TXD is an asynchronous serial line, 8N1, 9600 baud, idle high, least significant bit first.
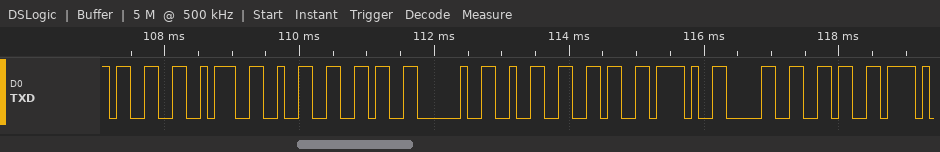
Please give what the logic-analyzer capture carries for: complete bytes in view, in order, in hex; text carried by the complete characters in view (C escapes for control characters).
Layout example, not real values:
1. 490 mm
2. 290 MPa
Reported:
1. 0x33 0x3A 0x32 0x36 0x20 0x32 0x36 0x2F 0x30 0x36
2. "3:26 26/06"
